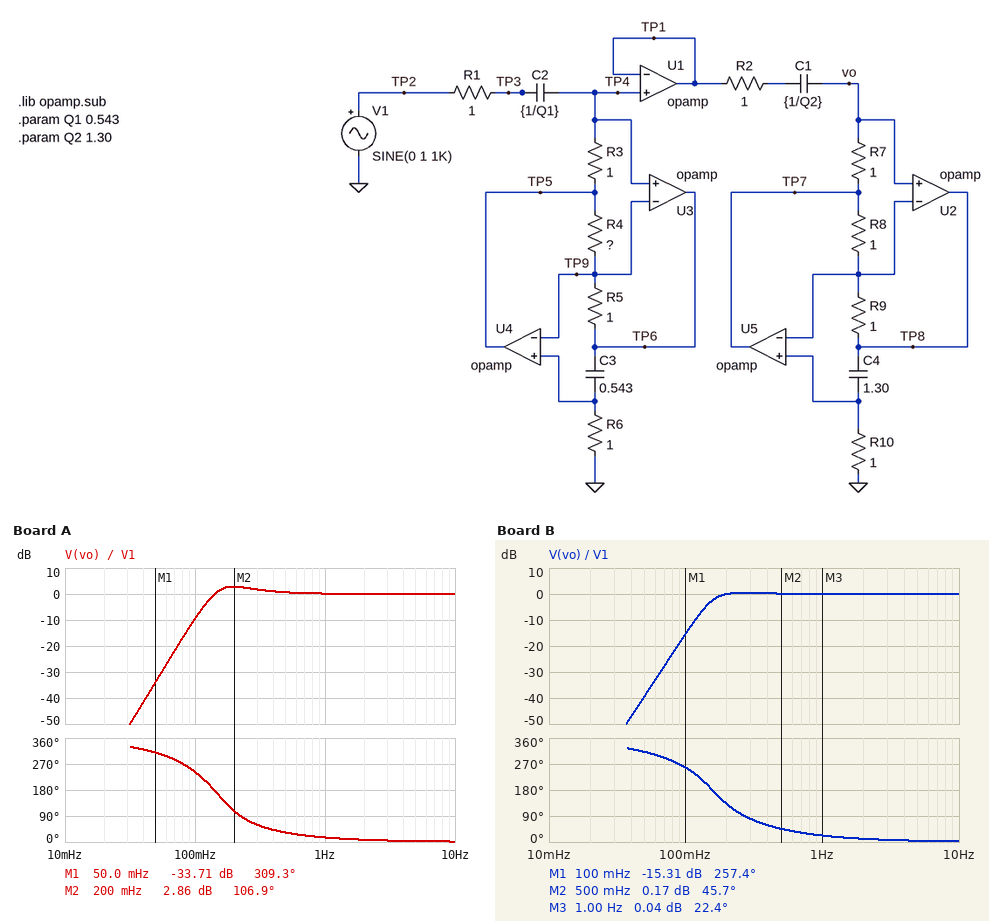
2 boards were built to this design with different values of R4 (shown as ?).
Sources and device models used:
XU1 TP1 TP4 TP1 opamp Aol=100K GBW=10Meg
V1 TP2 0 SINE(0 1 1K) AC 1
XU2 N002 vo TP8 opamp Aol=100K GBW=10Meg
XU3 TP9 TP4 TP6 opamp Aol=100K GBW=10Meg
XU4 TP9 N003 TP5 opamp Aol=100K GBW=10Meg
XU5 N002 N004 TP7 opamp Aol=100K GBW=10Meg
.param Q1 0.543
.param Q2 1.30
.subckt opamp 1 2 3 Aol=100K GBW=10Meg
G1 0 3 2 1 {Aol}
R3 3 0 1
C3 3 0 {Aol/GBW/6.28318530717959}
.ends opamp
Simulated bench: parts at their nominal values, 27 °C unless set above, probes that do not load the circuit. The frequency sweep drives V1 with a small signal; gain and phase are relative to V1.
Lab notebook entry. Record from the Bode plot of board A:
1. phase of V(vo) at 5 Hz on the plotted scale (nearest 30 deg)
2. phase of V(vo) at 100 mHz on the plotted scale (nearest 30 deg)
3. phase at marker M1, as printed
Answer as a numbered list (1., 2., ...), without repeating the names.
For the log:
1. 0 deg
2. 240 deg
3. 309.3 deg
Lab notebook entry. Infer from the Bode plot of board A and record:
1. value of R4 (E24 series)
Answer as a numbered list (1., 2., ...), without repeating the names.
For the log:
1. 0.51 Ω
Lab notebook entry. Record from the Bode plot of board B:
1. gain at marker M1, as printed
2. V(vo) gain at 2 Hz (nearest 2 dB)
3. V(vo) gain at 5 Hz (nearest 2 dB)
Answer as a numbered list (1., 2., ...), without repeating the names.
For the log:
1. -15.31 dB
2. 0 dB
3. 0 dB
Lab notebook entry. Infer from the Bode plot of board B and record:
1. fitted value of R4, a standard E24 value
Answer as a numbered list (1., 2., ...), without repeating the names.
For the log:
1. 0.91 Ω
